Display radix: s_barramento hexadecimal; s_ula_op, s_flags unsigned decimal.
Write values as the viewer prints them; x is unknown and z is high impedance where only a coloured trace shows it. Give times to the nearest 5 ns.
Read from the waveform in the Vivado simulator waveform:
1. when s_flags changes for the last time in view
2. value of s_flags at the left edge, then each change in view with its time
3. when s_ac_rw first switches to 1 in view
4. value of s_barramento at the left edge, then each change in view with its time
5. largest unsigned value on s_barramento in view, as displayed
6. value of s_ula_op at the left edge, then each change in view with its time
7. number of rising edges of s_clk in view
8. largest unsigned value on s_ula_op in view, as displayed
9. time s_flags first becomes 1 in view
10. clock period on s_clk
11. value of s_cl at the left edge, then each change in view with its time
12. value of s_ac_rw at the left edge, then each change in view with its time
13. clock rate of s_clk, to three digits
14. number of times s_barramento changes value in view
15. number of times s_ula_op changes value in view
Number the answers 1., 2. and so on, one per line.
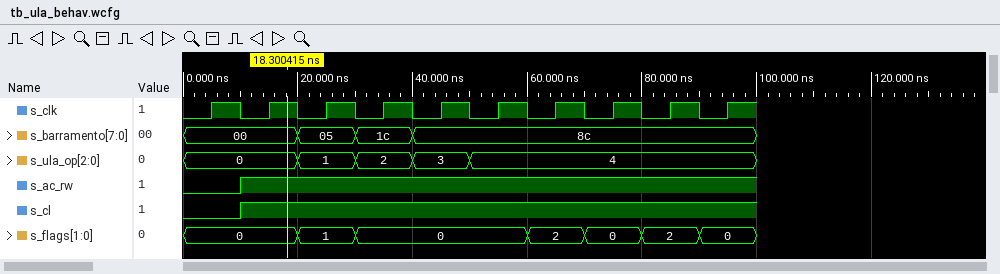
1. 90 ns
2. 0, 1 at 20 ns, 0 at 30 ns, 2 at 60 ns, 0 at 70 ns, 2 at 80 ns, 0 at 90 ns
3. 10 ns
4. 00, 05 at 20 ns, 1c at 30 ns, 8c at 40 ns
5. 8c
6. 0, 1 at 20 ns, 2 at 30 ns, 3 at 40 ns, 4 at 50 ns
7. 10
8. 4
9. 20 ns
10. 10 ns
11. 0, 1 at 10 ns
12. 0, 1 at 10 ns
13. 100 MHz
14. 3
15. 4
